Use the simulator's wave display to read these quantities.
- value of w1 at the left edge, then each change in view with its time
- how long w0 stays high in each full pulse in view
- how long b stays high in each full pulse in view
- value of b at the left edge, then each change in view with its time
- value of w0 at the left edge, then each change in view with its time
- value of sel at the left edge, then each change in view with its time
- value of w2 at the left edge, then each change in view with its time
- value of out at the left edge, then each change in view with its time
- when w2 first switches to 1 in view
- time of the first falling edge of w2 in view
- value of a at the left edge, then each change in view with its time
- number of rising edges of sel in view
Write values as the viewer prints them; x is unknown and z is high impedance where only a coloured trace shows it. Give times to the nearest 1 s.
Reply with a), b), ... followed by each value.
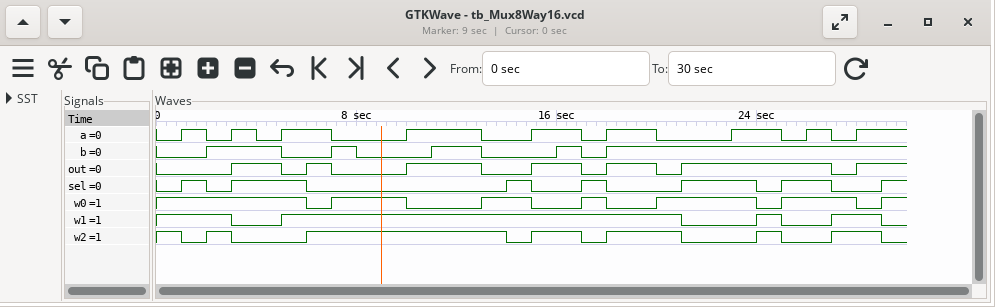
a) 1, 0 at 3 s, 1 at 5 s, 0 at 21 s, 1 at 24 s, 0 at 25 s, 1 at 27 s, 0 at 29 s
b) 3 s, 2 s, 1 s, 4 s, 3 s
c) 3 s, 1 s, 2 s, 1 s
d) 0, 1 at 2 s, 0 at 5 s, 1 at 7 s, 0 at 8 s, 1 at 11 s, 0 at 13 s, 1 at 16 s, 0 at 17 s, 1 at 18 s
e) 1, 0 at 6 s, 1 at 7 s, 0 at 10 s, 1 at 13 s, 0 at 15 s, 1 at 17 s, 0 at 18 s, 1 at 20 s, 0 at 24 s, 1 at 25 s, 0 at 28 s, 1 at 29 s
f) 0, 1 at 1 s, 0 at 2 s, 1 at 3 s, 0 at 6 s, 1 at 14 s, 0 at 15 s, 1 at 17 s, 0 at 18 s, 1 at 21 s, 0 at 24 s, 1 at 25 s, 0 at 27 s, 1 at 29 s
g) 1, 0 at 1 s, 1 at 2 s, 0 at 3 s, 1 at 6 s, 0 at 14 s, 1 at 15 s, 0 at 17 s, 1 at 18 s, 0 at 21 s, 1 at 24 s, 0 at 25 s, 1 at 27 s, 0 at 29 s
h) 0, 1 at 3 s, 0 at 5 s, 1 at 6 s, 0 at 7 s, 1 at 10 s, 0 at 13 s, 1 at 15 s, 0 at 17 s, 1 at 18 s, 0 at 20 s, 1 at 21 s, 0 at 27 s, 1 at 28 s
i) 2 s
j) 1 s
k) 0, 1 at 1 s, 0 at 2 s, 1 at 3 s, 0 at 4 s, 1 at 5 s, 0 at 7 s, 1 at 10 s, 0 at 13 s, 1 at 15 s, 0 at 17 s, 1 at 18 s, 0 at 20 s, 1 at 23 s, 0 at 25 s, 1 at 26 s, 0 at 27 s, 1 at 28 s
l) 7
